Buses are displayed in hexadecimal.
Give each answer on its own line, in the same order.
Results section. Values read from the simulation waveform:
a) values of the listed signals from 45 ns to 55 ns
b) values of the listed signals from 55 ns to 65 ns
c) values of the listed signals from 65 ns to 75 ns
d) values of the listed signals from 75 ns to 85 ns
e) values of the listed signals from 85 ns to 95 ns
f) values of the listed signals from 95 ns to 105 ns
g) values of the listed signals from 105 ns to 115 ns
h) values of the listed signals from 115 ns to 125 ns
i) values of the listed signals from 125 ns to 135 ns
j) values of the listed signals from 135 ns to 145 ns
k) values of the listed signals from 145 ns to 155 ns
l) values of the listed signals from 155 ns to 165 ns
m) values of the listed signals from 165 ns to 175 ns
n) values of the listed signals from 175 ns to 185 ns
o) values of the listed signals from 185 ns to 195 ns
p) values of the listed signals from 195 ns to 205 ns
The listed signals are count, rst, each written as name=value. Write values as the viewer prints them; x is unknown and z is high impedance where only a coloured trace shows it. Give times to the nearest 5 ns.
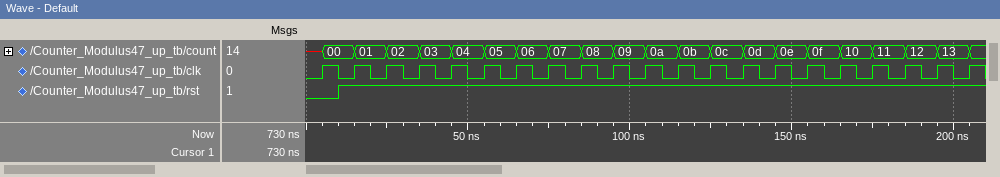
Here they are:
count=04, rst=1
count=05, rst=1
count=06, rst=1
count=07, rst=1
count=08, rst=1
count=09, rst=1
count=0a, rst=1
count=0b, rst=1
count=0c, rst=1
count=0d, rst=1
count=0e, rst=1
count=0f, rst=1
count=10, rst=1
count=11, rst=1
count=12, rst=1
count=13, rst=1
